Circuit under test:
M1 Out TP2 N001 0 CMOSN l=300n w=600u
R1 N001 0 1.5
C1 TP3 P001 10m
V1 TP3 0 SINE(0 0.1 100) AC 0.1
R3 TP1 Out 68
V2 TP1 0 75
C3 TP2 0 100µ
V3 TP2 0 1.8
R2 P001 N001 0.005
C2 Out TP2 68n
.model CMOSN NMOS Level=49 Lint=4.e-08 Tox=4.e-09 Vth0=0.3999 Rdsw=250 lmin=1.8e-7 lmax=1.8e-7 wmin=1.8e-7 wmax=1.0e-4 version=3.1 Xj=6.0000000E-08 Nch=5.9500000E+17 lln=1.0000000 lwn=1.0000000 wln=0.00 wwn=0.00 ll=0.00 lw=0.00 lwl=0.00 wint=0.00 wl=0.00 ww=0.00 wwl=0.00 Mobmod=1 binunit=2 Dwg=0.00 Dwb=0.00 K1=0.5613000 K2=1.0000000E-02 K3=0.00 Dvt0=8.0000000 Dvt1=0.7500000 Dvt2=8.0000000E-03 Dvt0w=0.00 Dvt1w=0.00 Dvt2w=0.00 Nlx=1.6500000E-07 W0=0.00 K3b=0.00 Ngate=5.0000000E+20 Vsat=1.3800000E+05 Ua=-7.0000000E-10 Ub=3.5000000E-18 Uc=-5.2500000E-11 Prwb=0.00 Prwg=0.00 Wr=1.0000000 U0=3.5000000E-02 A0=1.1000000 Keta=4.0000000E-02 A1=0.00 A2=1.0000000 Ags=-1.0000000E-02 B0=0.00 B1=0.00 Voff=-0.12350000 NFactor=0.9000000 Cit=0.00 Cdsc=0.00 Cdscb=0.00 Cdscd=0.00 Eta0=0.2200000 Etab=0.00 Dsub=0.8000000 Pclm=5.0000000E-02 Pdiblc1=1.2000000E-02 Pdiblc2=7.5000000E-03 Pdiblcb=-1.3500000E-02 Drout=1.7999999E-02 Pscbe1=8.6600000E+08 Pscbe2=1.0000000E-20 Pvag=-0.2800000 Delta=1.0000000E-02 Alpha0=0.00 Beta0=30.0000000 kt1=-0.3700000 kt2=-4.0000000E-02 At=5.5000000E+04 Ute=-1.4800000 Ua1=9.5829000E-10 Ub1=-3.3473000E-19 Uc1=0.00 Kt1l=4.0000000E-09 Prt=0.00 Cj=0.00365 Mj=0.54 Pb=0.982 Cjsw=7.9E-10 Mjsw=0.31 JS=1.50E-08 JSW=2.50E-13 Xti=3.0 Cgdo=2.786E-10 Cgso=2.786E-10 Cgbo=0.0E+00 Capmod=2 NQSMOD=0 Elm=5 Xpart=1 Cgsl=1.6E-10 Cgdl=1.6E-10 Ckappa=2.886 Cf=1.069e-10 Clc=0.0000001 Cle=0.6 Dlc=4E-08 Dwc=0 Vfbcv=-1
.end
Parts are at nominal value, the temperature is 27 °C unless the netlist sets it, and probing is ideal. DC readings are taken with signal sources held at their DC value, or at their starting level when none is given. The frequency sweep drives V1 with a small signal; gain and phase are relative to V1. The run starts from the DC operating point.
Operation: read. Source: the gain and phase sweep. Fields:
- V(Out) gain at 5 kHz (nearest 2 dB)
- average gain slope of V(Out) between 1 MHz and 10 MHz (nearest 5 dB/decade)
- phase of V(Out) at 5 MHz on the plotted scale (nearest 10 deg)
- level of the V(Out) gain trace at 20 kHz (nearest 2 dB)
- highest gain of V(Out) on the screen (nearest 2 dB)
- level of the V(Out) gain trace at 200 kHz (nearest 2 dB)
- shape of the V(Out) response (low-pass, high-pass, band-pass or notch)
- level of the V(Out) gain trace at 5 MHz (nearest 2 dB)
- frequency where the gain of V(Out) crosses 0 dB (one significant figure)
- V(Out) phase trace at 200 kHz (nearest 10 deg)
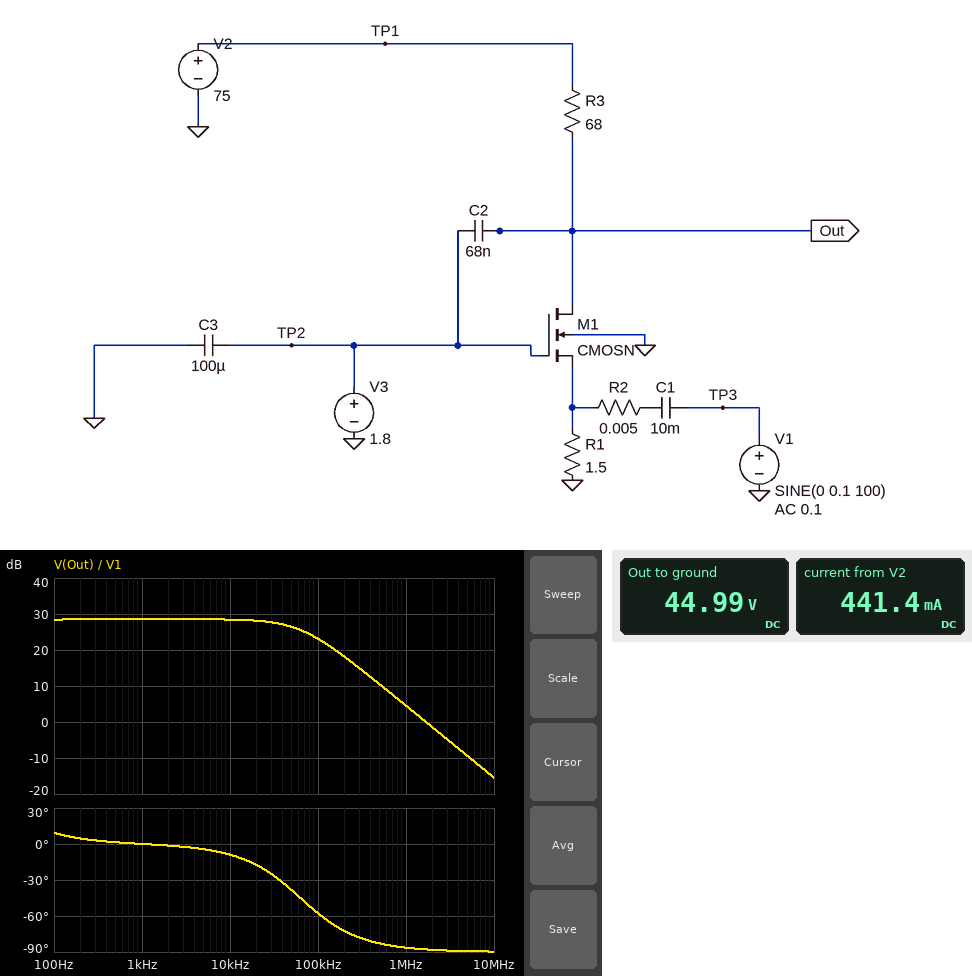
28 dB
-20 dB/decade
-90 deg
28 dB
28 dB
18 dB
low-pass
-10 dB
2 MHz
-70 deg
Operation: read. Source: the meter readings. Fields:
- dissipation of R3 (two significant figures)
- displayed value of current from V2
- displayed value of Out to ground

13 W
441.4 mA
44.99 V
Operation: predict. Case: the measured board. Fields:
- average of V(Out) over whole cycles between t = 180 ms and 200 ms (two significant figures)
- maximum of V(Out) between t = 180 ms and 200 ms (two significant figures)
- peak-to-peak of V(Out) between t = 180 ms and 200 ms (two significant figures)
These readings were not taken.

45 V
48 V
5.3 V
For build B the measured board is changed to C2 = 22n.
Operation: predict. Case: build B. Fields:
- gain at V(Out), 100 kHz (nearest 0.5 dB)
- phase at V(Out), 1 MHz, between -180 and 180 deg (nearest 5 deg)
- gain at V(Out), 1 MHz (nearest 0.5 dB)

27.5 dB
-80 deg
14.0 dB
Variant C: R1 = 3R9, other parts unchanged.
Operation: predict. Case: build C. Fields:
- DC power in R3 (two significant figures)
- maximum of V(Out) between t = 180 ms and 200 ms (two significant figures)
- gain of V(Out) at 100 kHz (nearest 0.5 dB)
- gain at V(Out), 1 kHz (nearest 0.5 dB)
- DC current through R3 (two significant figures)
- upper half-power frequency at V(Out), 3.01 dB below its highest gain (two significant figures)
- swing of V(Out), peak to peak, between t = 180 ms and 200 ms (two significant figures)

4.6 W
62 V
27.0 dB
33.0 dB
260 mA
57 kHz
8.8 V
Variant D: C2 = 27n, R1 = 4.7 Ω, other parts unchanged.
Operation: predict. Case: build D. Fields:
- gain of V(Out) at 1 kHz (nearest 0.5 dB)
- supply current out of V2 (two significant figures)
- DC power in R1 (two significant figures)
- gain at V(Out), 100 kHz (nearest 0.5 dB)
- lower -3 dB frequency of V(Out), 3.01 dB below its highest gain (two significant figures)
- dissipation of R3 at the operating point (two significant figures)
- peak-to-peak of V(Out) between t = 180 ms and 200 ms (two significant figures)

33.5 dB
230 mA
240 mW
32.0 dB
15 Hz
3.5 W
9.4 V
